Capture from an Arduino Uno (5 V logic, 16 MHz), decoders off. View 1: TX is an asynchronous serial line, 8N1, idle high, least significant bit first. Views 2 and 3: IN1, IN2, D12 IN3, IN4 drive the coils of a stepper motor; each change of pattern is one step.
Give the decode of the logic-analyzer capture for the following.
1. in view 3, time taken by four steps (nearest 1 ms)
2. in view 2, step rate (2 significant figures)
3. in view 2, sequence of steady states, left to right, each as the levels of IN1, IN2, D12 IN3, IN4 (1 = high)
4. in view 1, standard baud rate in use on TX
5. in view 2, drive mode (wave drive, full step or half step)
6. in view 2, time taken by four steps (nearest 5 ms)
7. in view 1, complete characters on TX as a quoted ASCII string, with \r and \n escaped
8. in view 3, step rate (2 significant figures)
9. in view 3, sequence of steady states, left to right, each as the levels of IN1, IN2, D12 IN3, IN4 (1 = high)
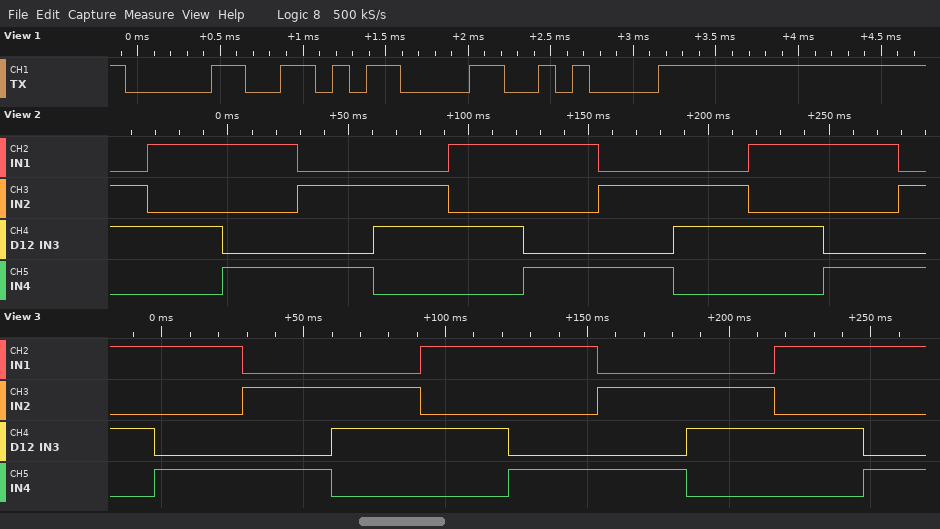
125 ms
32 steps/s
0110 1010 1001 0101 0110 1010 1001 0101 0110 1010 1001 0101
9600 baud
full step
125 ms
"0\r\n"
32 steps/s
1010 1001 0101 0110 1010 1001 0101 0110 1010 1001
